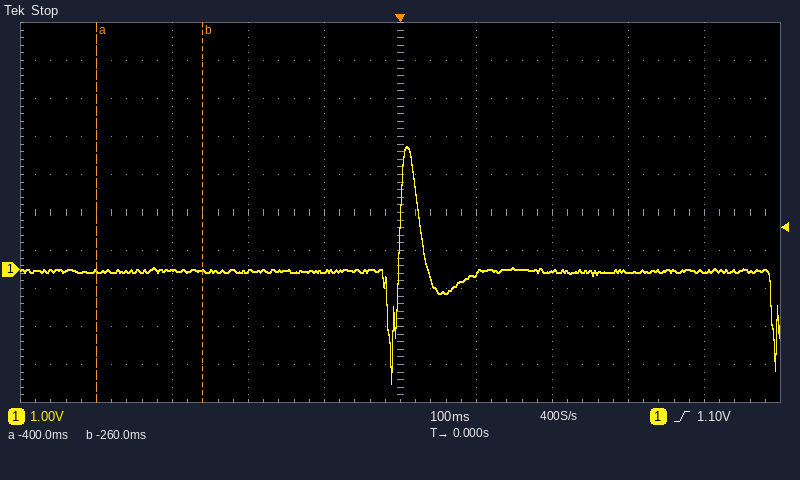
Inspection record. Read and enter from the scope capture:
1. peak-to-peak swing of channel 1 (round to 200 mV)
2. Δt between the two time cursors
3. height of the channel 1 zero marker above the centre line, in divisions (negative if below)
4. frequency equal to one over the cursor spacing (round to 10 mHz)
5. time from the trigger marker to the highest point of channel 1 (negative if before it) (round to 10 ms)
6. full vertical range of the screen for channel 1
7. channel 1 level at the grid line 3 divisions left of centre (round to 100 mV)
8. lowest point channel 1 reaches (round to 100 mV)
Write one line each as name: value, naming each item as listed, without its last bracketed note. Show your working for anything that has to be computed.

peak-to-peak swing of channel 1: 6.2 V
Δt between the two time cursors: -260 ms − (-400 ms) = 140 ms
height of the channel 1 zero marker above the centre line, in divisions: -1.5 div
frequency equal to one over the cursor spacing: 1 / 140 ms ≈ 7.14 Hz
time from the trigger marker to the highest point of channel 1 (negative if before it): +10 ms
full vertical range of the screen for channel 1: 10 V
channel 1 level at the grid line 3 divisions left of centre: 0.0 V
lowest point channel 1 reaches: -3.0 V
